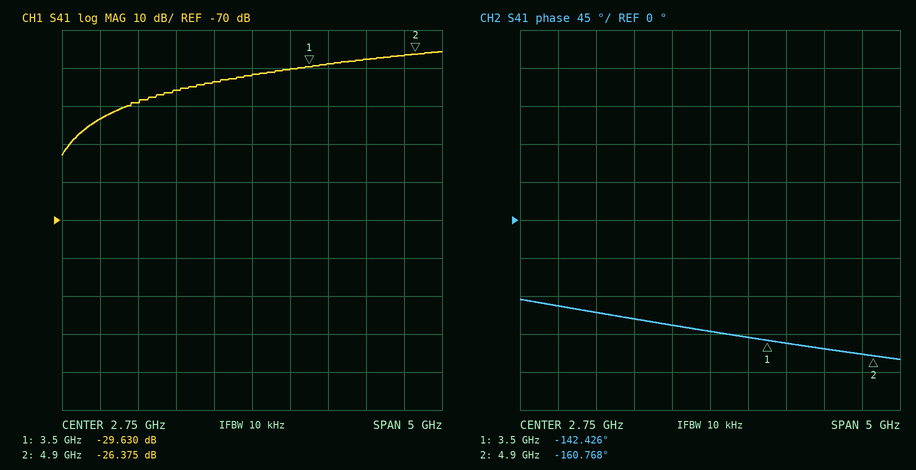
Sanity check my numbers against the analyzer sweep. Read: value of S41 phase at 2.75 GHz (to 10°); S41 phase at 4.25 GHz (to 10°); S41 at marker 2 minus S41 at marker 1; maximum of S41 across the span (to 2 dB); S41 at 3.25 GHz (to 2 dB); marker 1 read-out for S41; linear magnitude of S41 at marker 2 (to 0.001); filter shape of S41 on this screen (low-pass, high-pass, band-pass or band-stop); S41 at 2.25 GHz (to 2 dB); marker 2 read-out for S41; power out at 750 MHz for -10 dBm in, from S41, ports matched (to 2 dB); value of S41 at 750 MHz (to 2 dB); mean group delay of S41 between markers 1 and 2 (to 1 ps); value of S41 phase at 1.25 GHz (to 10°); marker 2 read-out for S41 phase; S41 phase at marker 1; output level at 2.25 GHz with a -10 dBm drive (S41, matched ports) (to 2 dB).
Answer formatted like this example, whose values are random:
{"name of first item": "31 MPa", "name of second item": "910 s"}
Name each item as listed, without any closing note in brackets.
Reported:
{"value of S41 phase at 2.75 GHz": "-130°", "S41 phase at 4.25 GHz": "-150°", "S41 at marker 2 minus S41 at marker 1": "3.255 dB", "maximum of S41 across the span": "-26 dB", "S41 at 3.25 GHz": "-30 dB", "marker 1 read-out for S41": "-29.630 dB", "linear magnitude of S41 at marker 2": "0.048", "filter shape of S41 on this screen": "high-pass", "S41 at 2.25 GHz": "-34 dB", "marker 2 read-out for S41": "-26.375 dB", "power out at 750 MHz for -10 dBm in, from S41, ports matched": "-54 dBm", "value of S41 at 750 MHz": "-44 dB", "mean group delay of S41 between markers 1 and 2": "36 ps", "value of S41 phase at 1.25 GHz": "-110°", "marker 2 read-out for S41 phase": "-160.768°", "S41 phase at marker 1": "-142.426°", "output level at 2.25 GHz with a -10 dBm drive (S41, matched ports)": "-44 dBm"}
